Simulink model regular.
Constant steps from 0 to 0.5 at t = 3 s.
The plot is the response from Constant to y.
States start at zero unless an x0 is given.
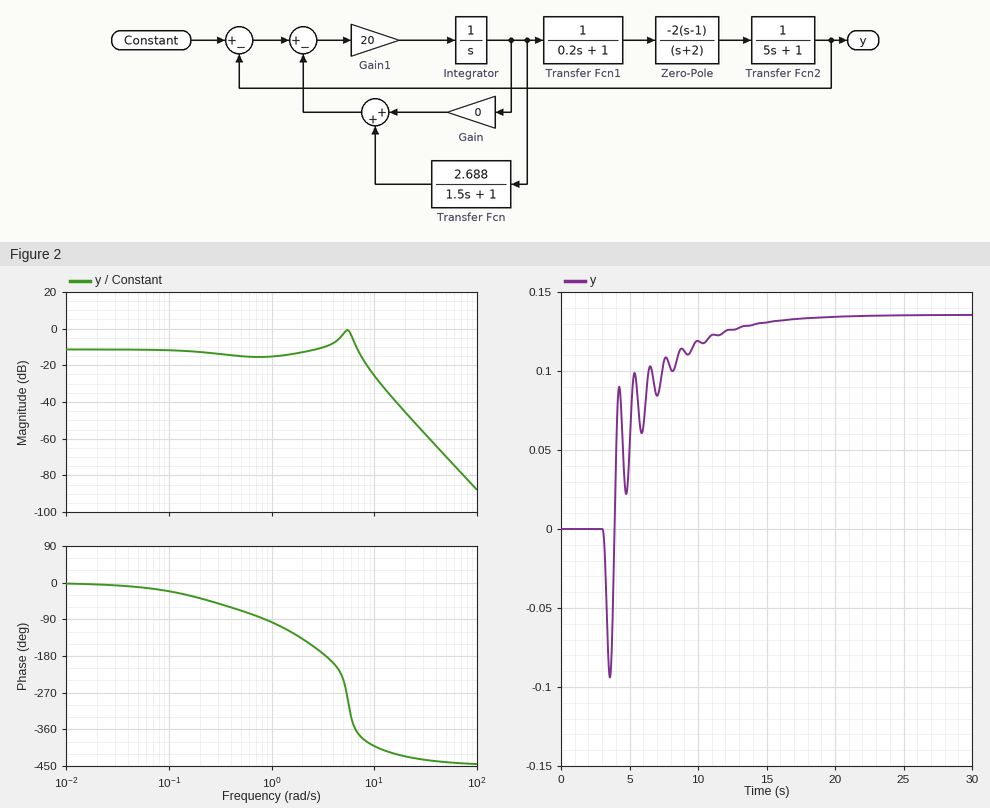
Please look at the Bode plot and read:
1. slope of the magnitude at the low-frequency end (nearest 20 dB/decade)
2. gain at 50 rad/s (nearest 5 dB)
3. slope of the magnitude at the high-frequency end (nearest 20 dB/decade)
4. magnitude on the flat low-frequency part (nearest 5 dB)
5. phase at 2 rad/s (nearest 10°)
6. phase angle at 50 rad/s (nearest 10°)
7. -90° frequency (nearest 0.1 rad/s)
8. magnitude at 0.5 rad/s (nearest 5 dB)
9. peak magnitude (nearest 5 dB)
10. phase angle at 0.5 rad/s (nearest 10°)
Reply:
0 dB/decade
-70 dB
-60 dB/decade
-10 dB
-140°
-440°
0.9 rad/s
-15 dB
0 dB
-70°
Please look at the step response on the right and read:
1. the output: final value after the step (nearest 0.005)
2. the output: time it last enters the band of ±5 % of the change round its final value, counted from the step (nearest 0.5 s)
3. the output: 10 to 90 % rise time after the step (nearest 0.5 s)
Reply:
0.135
11.0 s
7.0 s
